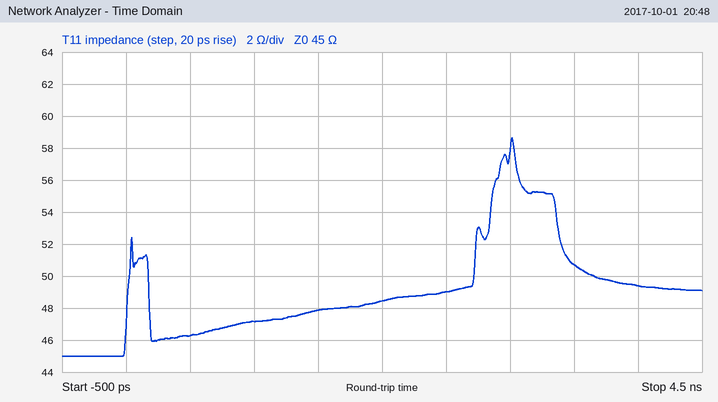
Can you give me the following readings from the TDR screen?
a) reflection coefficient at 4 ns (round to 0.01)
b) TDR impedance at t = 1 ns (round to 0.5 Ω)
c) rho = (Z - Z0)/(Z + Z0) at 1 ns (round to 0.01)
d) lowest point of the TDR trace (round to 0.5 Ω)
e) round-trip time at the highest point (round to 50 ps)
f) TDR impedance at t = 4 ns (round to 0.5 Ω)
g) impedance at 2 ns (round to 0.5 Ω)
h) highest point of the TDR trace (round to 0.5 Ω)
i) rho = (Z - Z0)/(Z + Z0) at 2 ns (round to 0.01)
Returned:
+0.05
47.0 Ω
+0.02
45.0 Ω
3.00 ns
49.5 Ω
48.5 Ω
58.5 Ω
+0.04
